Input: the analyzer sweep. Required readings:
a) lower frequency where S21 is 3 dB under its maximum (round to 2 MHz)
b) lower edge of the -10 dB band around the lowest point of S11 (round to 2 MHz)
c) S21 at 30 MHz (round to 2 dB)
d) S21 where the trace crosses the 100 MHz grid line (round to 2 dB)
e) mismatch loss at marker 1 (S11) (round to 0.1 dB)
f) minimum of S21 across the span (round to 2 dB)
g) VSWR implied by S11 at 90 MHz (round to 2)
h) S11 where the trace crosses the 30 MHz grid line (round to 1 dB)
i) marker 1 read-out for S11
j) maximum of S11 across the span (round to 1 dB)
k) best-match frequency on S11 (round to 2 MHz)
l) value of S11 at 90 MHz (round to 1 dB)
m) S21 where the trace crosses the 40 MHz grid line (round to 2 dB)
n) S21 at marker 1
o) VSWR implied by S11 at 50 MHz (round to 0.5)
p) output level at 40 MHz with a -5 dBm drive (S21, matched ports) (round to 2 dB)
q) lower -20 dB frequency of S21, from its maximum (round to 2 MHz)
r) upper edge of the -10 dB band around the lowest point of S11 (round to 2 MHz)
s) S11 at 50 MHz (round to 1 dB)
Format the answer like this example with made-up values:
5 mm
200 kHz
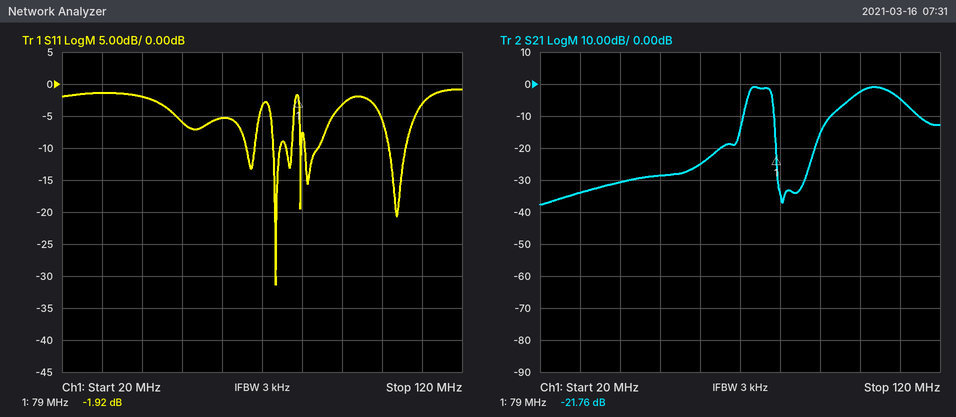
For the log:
72 MHz
72 MHz
-34 dB
-2 dB
4.5 dB
-38 dB
6
-1 dB
-1.92 dB
-1 dB
74 MHz
-3 dB
-30 dB
-21.76 dB
3.0
-36 dBm
64 MHz
74 MHz
-6 dB
